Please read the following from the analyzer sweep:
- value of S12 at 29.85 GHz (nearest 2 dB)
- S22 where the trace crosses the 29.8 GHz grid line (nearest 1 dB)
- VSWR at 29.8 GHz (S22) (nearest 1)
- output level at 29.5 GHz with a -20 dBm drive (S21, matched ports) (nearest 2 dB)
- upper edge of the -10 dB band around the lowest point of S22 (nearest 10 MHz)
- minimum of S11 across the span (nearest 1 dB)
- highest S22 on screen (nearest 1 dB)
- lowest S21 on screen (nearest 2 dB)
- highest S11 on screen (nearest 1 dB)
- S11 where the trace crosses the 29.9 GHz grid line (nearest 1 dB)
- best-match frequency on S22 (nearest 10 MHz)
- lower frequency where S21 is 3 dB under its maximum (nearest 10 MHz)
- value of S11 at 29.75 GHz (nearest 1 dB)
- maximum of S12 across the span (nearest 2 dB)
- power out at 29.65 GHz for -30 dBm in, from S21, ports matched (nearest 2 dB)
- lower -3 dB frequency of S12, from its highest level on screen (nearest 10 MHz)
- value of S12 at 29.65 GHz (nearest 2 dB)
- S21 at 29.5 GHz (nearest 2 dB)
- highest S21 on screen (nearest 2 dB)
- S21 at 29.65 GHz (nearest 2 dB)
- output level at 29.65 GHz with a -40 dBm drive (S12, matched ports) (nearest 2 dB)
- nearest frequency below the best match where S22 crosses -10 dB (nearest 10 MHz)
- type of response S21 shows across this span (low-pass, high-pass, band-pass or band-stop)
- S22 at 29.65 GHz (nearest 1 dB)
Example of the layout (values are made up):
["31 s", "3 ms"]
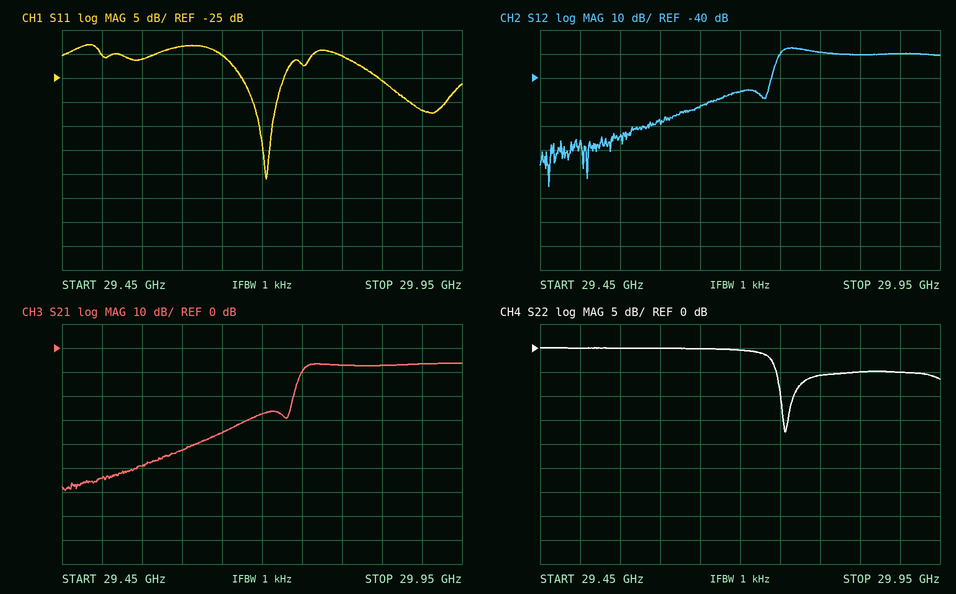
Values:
["-30 dB", "-6 dB", "3", "-74 dBm", "29.77 GHz", "-46 dB", "0 dB", "-60 dB", "-18 dB", "-32 dB", "29.76 GHz", "29.75 GHz", "-22 dB", "-28 dB", "-66 dBm", "29.75 GHz", "-52 dB", "-54 dB", "-6 dB", "-36 dB", "-92 dBm", "29.75 GHz", "high-pass", "0 dB"]
